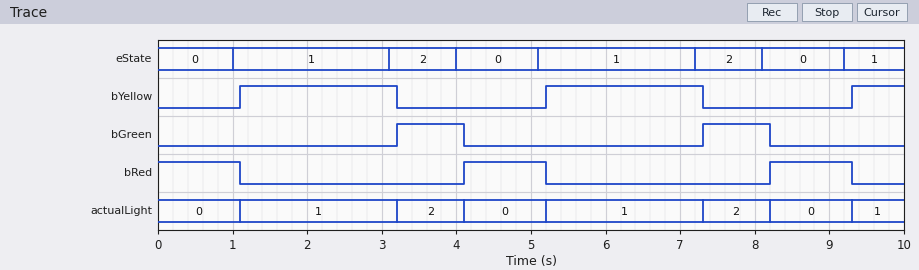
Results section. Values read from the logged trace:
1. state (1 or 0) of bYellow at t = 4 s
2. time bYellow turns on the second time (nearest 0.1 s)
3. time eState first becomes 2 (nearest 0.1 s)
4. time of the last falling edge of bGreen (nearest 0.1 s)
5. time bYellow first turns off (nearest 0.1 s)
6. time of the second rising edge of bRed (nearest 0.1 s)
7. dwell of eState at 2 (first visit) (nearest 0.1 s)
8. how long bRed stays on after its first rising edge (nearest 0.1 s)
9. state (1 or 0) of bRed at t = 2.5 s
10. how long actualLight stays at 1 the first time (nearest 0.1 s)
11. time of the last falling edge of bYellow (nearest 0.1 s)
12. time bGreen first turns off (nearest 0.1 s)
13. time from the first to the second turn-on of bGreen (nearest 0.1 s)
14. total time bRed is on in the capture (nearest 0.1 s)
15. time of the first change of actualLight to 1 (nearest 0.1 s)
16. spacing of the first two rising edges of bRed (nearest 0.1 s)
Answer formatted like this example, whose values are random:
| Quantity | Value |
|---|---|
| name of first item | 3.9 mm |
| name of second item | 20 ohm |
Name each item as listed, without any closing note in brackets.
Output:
| Quantity | Value |
|---|---|
| state (1 or 0) of bYellow at t = 4 s | 0 |
| time bYellow turns on the second time | 5.2 s |
| time eState first becomes 2 | 3.1 s |
| time of the last falling edge of bGreen | 8.2 s |
| time bYellow first turns off | 3.2 s |
| time of the second rising edge of bRed | 8.2 s |
| dwell of eState at 2 (first visit) | 0.9 s |
| how long bRed stays on after its first rising edge | 1.1 s |
| state (1 or 0) of bRed at t = 2.5 s | 0 |
| how long actualLight stays at 1 the first time | 2.1 s |
| time of the last falling edge of bYellow | 7.3 s |
| time bGreen first turns off | 4.1 s |
| time from the first to the second turn-on of bGreen | 4.1 s |
| total time bRed is on in the capture | 3.3 s |
| time of the first change of actualLight to 1 | 1.1 s |
| spacing of the first two rising edges of bRed | 4.1 s |
